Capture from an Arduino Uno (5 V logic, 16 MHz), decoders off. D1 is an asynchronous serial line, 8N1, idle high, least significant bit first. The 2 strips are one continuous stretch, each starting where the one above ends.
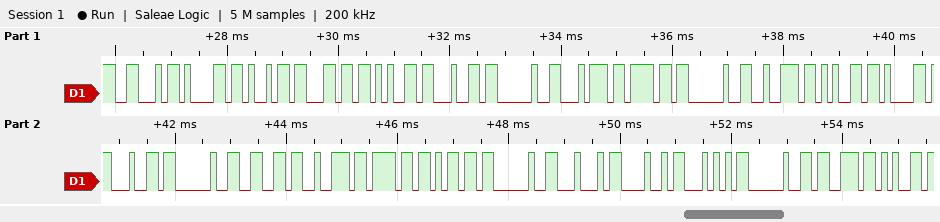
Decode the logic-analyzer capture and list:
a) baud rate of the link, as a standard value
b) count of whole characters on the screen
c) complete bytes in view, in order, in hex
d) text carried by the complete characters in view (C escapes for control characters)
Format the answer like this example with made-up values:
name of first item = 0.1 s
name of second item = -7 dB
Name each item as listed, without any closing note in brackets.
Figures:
baud rate of the link, as a standard value = 9600 baud
count of whole characters on the screen = 26
complete bytes in view, in order, in hex = 46 61 69 6C 65 64 20 74 6F 20 72 65 61 64 20 66 72 6F 6D 20 44 48 54 20 73 65
text carried by the complete characters in view = "Failed to read from DHT se"
